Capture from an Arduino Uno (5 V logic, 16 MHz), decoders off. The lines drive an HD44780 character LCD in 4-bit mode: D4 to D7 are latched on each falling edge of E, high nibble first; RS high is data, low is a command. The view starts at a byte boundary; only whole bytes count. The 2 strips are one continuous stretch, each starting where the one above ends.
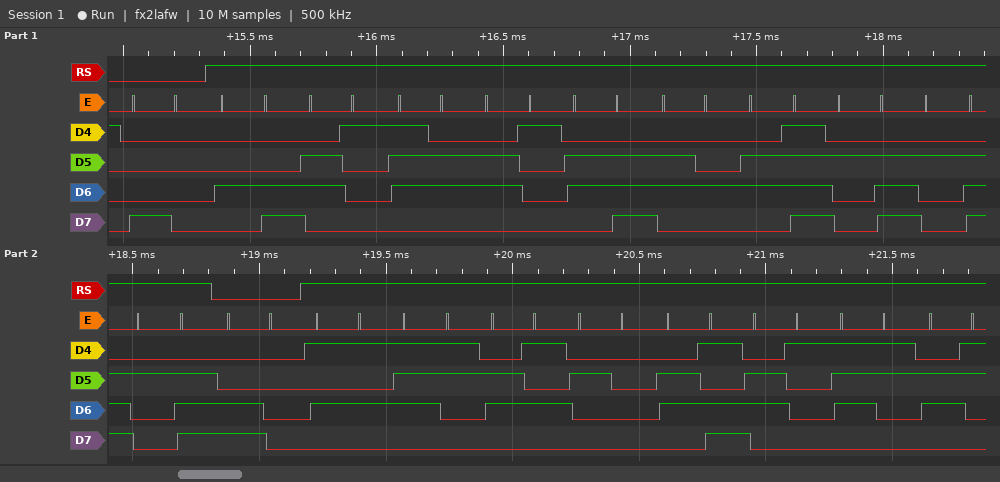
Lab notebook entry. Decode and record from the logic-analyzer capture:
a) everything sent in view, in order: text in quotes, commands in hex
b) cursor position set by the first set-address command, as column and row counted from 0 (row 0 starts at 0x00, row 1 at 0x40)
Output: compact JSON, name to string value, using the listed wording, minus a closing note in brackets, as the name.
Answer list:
{"everything sent in view, in order: text in quotes, commands in hex": "0x80 \"Lavando...\" 0xC0 \"Use masc\"", "cursor position set by the first set-address command, as column and row counted from 0": "column 0, row 0"}
